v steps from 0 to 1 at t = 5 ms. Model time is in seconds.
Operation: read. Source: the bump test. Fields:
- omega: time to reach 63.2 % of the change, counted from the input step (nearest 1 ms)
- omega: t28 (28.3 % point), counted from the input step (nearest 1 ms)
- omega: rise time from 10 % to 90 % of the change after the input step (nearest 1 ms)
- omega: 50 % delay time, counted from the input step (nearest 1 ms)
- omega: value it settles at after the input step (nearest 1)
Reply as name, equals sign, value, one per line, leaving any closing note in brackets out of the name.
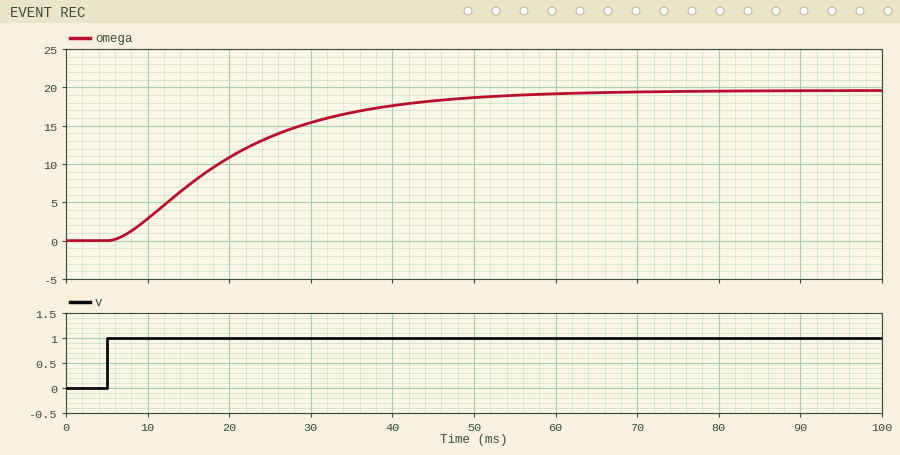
omega: time to reach 63.2 % of the change, counted from the input step = 18 ms
omega: t28 (28.3 % point), counted from the input step = 8 ms
omega: rise time from 10 % to 90 % of the change after the input step = 31 ms
omega: 50 % delay time, counted from the input step = 13 ms
omega: value it settles at after the input step = 20
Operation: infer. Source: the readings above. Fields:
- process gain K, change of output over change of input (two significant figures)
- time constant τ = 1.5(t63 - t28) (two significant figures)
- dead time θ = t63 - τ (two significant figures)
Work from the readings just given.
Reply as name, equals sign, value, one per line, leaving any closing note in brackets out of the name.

process gain K, change of output over change of input = 20
time constant τ = 1.5(t63 - t28) = 15 ms
dead time θ = t63 - τ = 3.0 ms
